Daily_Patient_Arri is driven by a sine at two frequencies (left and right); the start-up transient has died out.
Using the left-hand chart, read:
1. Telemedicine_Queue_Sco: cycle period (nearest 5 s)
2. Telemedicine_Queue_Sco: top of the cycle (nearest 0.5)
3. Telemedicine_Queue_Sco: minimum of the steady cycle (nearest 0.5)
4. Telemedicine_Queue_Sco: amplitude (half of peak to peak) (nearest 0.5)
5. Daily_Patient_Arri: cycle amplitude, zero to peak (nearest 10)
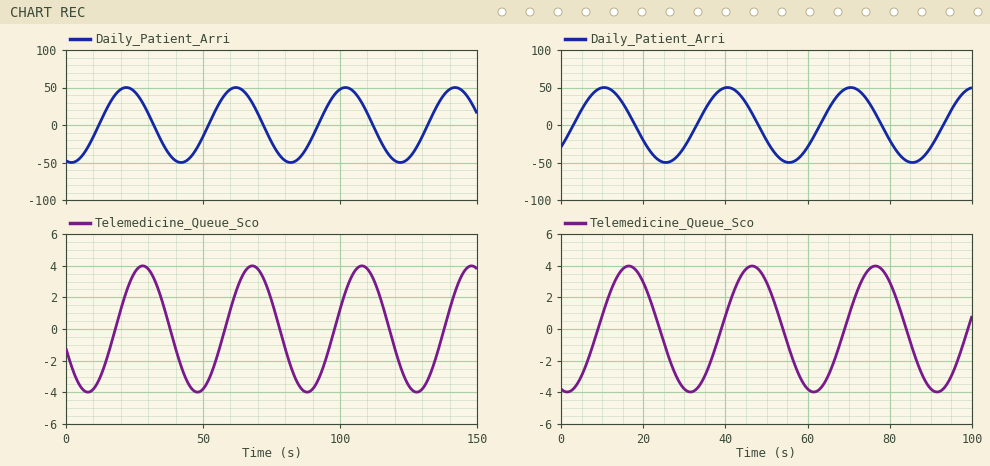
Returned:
40 s
4.0
-4.0
4.0
50
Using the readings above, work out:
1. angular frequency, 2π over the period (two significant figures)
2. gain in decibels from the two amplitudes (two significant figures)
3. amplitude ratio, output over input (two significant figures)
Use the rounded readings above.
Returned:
0.16 rad/s
-22 dB
0.080
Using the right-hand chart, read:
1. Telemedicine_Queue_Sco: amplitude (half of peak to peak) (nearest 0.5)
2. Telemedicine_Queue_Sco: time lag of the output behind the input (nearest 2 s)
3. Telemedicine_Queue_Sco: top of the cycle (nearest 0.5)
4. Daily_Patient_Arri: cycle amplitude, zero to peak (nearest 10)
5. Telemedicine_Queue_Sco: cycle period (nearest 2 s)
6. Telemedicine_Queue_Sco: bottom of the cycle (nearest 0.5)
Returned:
4.0
6 s
4.0
50
30 s
-4.0
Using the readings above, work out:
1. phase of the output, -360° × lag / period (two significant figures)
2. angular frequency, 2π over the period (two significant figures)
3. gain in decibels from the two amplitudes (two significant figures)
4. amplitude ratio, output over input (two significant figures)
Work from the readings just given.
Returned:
-72°
0.21 rad/s
-22 dB
0.080
